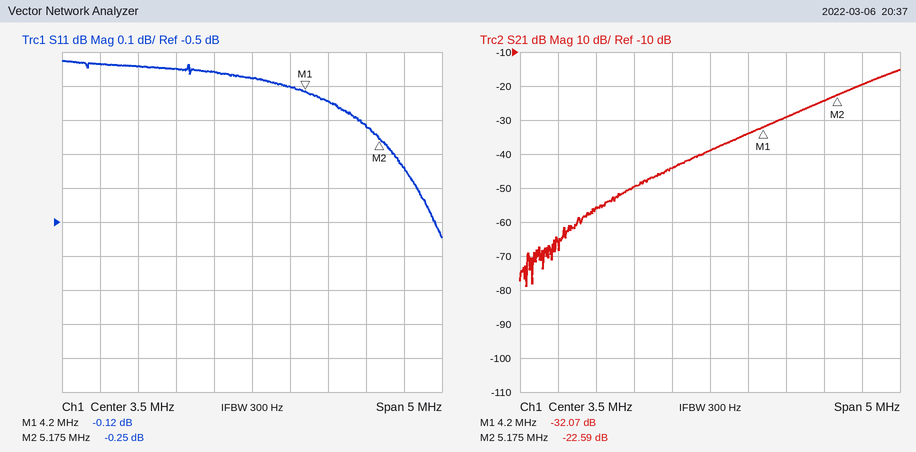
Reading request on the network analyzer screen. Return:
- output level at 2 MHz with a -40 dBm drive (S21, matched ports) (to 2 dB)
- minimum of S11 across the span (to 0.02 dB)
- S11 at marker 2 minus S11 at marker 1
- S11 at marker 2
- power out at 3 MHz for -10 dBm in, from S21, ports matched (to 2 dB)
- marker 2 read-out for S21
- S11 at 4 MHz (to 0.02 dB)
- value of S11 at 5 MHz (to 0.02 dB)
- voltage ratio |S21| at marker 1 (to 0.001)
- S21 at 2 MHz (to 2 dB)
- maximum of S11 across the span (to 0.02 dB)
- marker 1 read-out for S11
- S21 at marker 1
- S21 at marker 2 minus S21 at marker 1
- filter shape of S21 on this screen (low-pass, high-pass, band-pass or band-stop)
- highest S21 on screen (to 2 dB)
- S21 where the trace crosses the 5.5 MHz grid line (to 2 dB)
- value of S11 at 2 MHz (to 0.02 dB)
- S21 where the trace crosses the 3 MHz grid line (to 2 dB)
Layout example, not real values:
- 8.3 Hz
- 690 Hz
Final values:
- -96 dBm
- -0.54 dB
- -0.13 dB
- -0.25 dB
- -54 dBm
- -22.59 dB
- -0.10 dB
- -0.22 dB
- 0.025
- -56 dB
- -0.02 dB
- -0.12 dB
- -32.07 dB
- 9.48 dB
- high-pass
- -16 dB
- -20 dB
- -0.04 dB
- -44 dB
